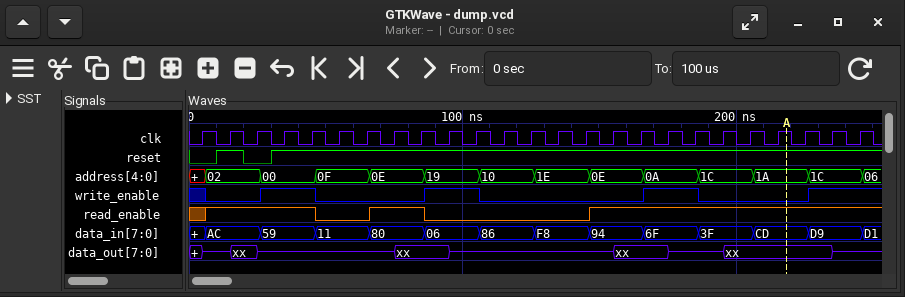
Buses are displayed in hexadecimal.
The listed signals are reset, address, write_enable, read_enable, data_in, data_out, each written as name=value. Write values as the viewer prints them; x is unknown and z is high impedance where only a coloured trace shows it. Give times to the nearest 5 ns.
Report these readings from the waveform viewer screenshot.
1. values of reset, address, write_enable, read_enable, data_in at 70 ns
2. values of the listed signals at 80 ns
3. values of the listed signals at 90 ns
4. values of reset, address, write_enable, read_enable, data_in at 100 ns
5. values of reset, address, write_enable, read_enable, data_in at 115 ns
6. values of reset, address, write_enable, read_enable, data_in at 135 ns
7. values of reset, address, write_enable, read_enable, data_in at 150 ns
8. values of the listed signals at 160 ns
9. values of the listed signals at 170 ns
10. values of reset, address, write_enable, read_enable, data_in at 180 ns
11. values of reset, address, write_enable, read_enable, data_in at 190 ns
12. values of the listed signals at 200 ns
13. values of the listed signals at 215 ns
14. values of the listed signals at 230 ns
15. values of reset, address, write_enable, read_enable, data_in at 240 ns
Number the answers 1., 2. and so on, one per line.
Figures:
1. reset=1, address=0E, write_enable=0, read_enable=1, data_in=80
2. reset=1, address=0E, write_enable=0, read_enable=1, data_in=80, data_out=xx
3. reset=1, address=19, write_enable=1, read_enable=0, data_in=06, data_out=xx
4. reset=1, address=19, write_enable=1, read_enable=0, data_in=06
5. reset=1, address=10, write_enable=0, read_enable=0, data_in=86
6. reset=1, address=1E, write_enable=0, read_enable=0, data_in=F8
7. reset=1, address=0E, write_enable=0, read_enable=1, data_in=94
8. reset=1, address=0E, write_enable=0, read_enable=1, data_in=94, data_out=xx
9. reset=1, address=0A, write_enable=1, read_enable=1, data_in=6F, data_out=xx
10. reset=1, address=0A, write_enable=1, read_enable=1, data_in=6F
11. reset=1, address=1C, write_enable=0, read_enable=1, data_in=3F
12. reset=1, address=1C, write_enable=0, read_enable=1, data_in=3F, data_out=xx
13. reset=1, address=1A, write_enable=0, read_enable=1, data_in=CD, data_out=xx
14. reset=1, address=1C, write_enable=1, read_enable=1, data_in=D9, data_out=xx
15. reset=1, address=1C, write_enable=1, read_enable=1, data_in=D9
